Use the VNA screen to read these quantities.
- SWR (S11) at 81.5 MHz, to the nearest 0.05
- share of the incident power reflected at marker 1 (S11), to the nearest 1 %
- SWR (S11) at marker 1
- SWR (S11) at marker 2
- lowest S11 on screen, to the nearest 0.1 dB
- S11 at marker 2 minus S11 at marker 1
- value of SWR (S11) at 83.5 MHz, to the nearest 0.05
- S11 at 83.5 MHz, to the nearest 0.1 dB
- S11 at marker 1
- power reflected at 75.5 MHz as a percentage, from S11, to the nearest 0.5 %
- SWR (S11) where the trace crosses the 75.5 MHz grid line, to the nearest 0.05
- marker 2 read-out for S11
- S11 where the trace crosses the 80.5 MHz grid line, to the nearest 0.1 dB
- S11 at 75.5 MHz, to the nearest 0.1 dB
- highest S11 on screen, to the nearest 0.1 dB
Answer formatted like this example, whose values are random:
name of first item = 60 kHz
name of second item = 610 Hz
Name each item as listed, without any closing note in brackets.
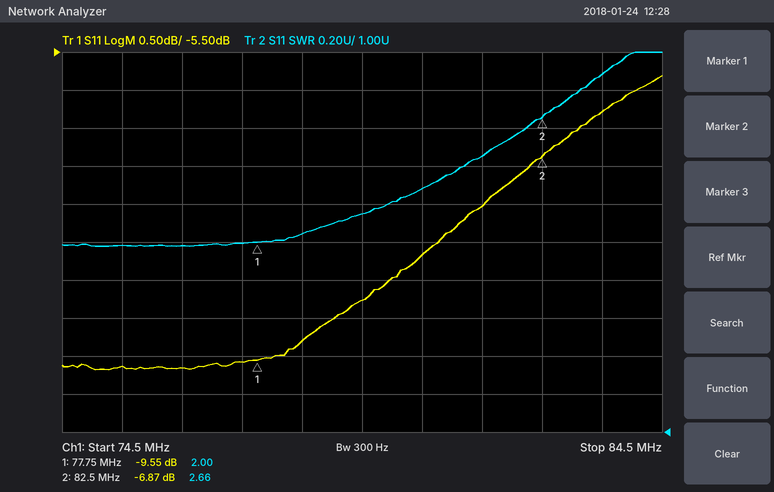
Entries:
SWR (S11) at 81.5 MHz, to the nearest 0.05 = 2.45
share of the incident power reflected at marker 1 (S11), to the nearest 1 % = 11 %
SWR (S11) at marker 1 = 2.00
SWR (S11) at marker 2 = 2.66
lowest S11 on screen, to the nearest 0.1 dB = -9.7 dB
S11 at marker 2 minus S11 at marker 1 = 2.68 dB
value of SWR (S11) at 83.5 MHz, to the nearest 0.05 = 2.90
S11 at 83.5 MHz, to the nearest 0.1 dB = -6.3 dB
S11 at marker 1 = -9.55 dB
power reflected at 75.5 MHz as a percentage, from S11, to the nearest 0.5 % = 11.0 %
SWR (S11) where the trace crosses the 75.5 MHz grid line, to the nearest 0.05 = 2.00
marker 2 read-out for S11 = -6.87 dB
S11 where the trace crosses the 80.5 MHz grid line, to the nearest 0.1 dB = -8.2 dB
S11 at 75.5 MHz, to the nearest 0.1 dB = -9.6 dB
highest S11 on screen, to the nearest 0.1 dB = -5.8 dB
